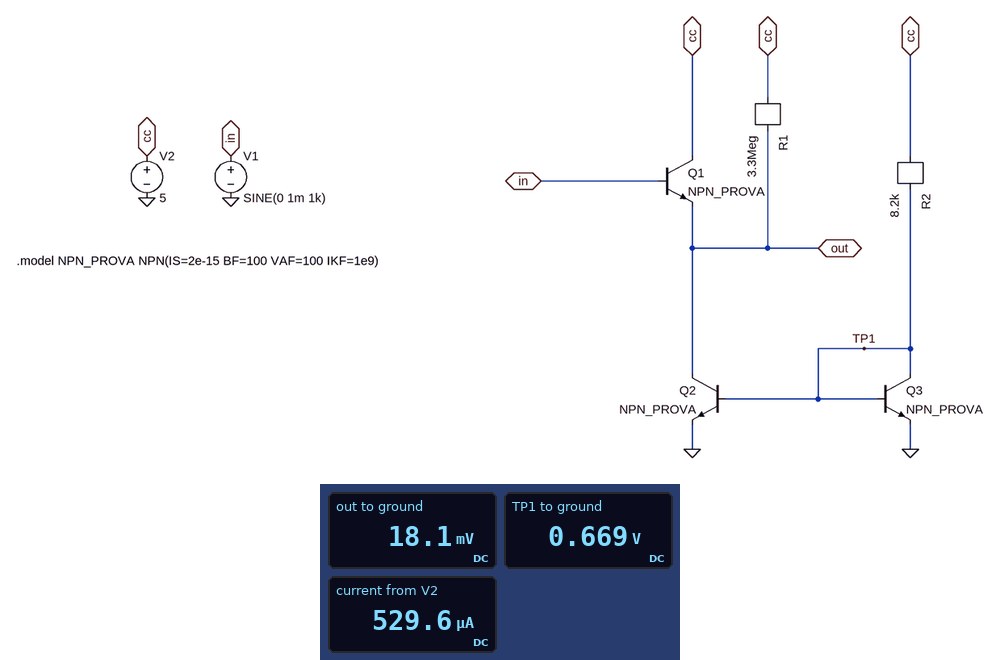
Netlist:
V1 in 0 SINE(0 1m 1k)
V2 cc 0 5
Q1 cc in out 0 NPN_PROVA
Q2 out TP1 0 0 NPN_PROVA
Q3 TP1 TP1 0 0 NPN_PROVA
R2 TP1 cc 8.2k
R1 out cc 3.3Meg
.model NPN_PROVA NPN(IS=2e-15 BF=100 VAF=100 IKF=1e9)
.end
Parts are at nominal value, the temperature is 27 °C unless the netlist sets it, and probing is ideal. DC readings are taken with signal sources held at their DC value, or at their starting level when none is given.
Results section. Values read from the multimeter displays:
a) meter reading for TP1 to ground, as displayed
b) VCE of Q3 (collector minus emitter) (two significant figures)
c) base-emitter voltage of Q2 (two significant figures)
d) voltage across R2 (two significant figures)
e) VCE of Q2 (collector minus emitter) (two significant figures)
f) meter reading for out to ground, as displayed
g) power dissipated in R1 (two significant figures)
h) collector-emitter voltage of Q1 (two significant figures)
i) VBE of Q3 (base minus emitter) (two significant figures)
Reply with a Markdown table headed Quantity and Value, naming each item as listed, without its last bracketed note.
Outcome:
| Quantity | Value |
|---|---|
| meter reading for TP1 to ground, as displayed | 0.669 V |
| VCE of Q3 (collector minus emitter) | 670 mV |
| base-emitter voltage of Q2 | 670 mV |
| voltage across R2 | 4.3 V |
| VCE of Q2 (collector minus emitter) | 18 mV |
| meter reading for out to ground, as displayed | 18.1 mV |
| power dissipated in R1 | 7.5 µW |
| collector-emitter voltage of Q1 | 5.0 V |
| VBE of Q3 (base minus emitter) | 670 mV |
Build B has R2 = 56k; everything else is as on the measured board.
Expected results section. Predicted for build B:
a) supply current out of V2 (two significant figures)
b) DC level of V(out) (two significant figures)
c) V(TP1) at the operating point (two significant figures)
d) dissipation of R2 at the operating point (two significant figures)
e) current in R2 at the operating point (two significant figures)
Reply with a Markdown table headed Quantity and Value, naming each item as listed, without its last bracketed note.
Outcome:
| Quantity | Value |
|---|---|
| supply current out of V2 | 80 µA |
| DC level of V(out) | 19 mV |
| V(TP1) at the operating point | 620 mV |
| dissipation of R2 at the operating point | 340 µW |
| current in R2 at the operating point | 78 µA |
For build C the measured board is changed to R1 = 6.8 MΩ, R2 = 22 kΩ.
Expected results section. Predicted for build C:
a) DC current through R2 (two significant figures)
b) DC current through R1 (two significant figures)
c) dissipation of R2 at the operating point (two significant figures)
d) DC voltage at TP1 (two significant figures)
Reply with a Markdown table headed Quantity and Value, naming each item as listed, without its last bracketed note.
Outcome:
| Quantity | Value |
|---|---|
| DC current through R2 | 200 µA |
| DC current through R1 | 730 nA |
| dissipation of R2 at the operating point | 860 µW |
| DC voltage at TP1 | 640 mV |
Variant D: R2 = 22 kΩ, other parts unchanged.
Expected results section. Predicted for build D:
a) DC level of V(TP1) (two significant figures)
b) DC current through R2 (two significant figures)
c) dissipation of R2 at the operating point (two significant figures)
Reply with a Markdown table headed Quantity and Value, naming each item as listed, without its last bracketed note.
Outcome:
| Quantity | Value |
|---|---|
| DC level of V(TP1) | 640 mV |
| DC current through R2 | 200 µA |
| dissipation of R2 at the operating point | 860 µW |
